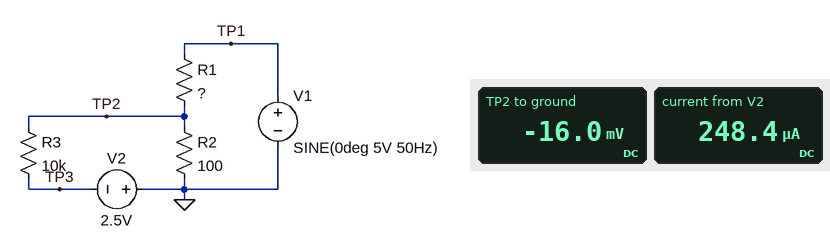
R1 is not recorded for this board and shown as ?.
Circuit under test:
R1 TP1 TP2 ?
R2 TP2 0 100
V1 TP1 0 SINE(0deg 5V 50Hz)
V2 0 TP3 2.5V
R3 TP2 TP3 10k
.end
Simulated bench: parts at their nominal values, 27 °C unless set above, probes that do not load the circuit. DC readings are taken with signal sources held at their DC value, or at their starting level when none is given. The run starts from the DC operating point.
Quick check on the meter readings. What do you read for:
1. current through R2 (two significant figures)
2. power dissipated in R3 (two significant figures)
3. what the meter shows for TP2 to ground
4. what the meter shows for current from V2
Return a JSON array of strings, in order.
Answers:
["160 µA", "620 µW", "-16.0 mV", "248.4 µA"]
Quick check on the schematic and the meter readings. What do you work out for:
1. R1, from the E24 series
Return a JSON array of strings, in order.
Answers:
["180 Ω"]
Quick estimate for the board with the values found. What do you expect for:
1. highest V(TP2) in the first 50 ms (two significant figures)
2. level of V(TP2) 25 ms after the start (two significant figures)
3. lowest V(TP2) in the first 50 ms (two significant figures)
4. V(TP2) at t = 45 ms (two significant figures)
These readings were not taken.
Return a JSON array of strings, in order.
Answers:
["1.8 V", "1.8 V", "-1.8 V", "1.8 V"]
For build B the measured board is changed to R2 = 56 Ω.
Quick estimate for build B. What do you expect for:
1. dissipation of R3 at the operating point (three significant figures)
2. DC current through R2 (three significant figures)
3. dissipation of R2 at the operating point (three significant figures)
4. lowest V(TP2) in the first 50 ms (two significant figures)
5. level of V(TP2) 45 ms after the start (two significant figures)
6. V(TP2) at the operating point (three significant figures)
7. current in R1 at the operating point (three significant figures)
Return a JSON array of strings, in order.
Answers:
["620 µW", "190 µA", "2.02 µW", "-1.2 V", "1.2 V", "-10.6 mV", "59.1 µA"]
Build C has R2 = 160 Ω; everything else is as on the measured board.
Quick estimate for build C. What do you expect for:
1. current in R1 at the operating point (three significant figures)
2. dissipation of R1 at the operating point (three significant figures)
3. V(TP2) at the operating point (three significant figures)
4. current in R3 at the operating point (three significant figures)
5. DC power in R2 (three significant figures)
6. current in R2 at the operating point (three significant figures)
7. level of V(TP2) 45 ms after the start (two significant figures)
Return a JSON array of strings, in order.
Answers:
["117 µA", "2.45 µW", "-21.0 mV", "248 µA", "2.76 µW", "131 µA", "2.3 V"]
